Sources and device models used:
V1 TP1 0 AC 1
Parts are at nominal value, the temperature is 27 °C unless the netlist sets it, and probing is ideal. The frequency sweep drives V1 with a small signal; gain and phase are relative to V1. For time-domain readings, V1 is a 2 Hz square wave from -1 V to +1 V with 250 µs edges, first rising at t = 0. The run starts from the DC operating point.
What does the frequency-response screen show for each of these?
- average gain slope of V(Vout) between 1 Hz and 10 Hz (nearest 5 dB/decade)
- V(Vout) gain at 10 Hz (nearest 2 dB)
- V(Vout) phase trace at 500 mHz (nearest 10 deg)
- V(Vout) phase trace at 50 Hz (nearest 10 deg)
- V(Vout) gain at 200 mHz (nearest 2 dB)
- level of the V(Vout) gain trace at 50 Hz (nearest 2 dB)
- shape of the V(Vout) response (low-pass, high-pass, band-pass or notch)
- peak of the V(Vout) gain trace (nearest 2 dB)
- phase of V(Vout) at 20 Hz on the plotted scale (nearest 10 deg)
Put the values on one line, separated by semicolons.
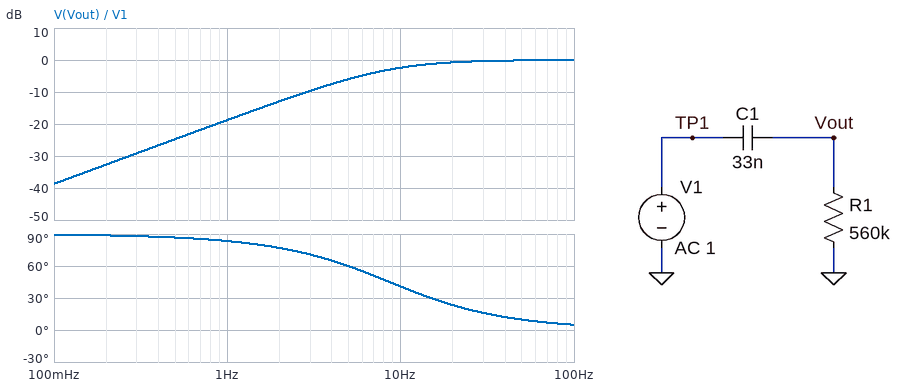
15 dB/decade; -2 dB; 90 deg; 10 deg; -32 dB; 0 dB; high-pass; 0 dB; 20 deg
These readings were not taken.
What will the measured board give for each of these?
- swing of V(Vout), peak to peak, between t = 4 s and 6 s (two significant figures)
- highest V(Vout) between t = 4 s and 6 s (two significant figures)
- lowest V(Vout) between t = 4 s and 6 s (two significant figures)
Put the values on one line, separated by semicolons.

4.0 V; 2.0 V; -2.0 V
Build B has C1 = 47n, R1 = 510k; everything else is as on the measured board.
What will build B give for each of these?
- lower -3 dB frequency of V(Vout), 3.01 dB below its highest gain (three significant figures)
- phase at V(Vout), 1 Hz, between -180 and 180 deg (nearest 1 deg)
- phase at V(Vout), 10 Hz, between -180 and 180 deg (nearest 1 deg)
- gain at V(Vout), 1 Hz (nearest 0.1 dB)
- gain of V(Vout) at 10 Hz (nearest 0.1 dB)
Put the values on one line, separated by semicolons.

6.64 Hz; 81 deg; 34 deg; -16.5 dB; -1.6 dB
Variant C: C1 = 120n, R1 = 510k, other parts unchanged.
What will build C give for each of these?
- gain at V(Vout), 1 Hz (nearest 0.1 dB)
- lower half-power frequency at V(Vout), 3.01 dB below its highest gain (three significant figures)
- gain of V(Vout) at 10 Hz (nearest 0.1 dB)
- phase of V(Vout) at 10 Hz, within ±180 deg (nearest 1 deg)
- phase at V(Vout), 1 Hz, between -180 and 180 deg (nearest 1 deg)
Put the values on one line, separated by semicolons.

-8.9 dB; 2.60 Hz; -0.3 dB; 15 deg; 69 deg
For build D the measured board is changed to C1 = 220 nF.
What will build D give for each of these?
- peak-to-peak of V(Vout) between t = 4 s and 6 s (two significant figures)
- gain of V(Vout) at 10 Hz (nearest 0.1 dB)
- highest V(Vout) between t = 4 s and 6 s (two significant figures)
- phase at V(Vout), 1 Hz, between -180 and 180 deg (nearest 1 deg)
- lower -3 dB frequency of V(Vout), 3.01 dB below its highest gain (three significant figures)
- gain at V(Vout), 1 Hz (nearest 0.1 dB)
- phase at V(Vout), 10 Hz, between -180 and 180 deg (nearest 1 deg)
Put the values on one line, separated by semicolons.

3.5 V; -0.1 dB; 1.8 V; 52 deg; 1.29 Hz; -4.3 dB; 7 deg
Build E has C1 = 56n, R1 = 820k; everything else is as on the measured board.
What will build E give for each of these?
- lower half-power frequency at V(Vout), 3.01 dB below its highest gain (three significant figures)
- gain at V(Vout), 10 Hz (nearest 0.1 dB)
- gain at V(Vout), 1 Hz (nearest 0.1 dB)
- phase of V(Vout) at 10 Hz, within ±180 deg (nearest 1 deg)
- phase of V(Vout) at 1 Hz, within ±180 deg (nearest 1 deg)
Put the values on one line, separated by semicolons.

3.47 Hz; -0.5 dB; -11.1 dB; 19 deg; 74 deg
